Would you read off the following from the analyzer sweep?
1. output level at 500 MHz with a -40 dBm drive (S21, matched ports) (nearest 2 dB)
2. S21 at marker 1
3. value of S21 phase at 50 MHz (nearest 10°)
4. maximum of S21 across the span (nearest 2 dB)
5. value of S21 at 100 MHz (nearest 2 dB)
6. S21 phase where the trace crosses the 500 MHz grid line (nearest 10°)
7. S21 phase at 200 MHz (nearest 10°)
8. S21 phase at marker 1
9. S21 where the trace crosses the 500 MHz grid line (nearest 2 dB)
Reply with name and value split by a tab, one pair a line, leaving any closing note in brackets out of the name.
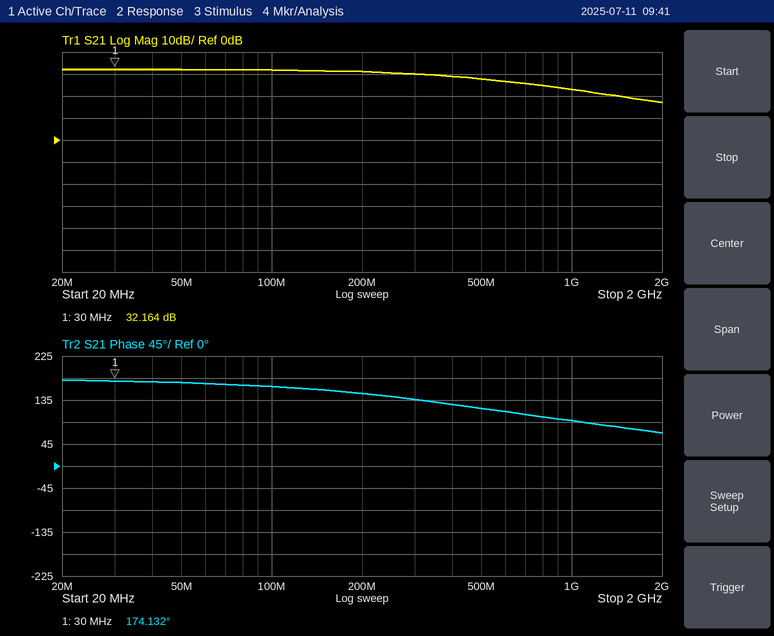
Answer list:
output level at 500 MHz with a -40 dBm drive (S21, matched ports)	-12 dBm
S21 at marker 1	32.164 dB
value of S21 phase at 50 MHz	170°
maximum of S21 across the span	32 dB
value of S21 at 100 MHz	32 dB
S21 phase where the trace crosses the 500 MHz grid line	120°
S21 phase at 200 MHz	150°
S21 phase at marker 1	174.132°
S21 where the trace crosses the 500 MHz grid line	28 dB
